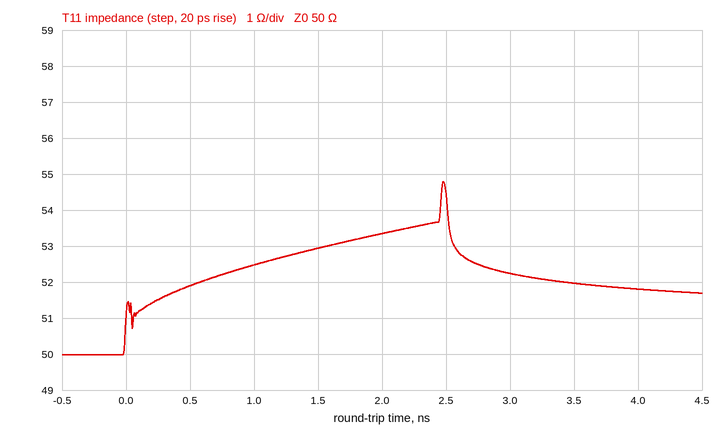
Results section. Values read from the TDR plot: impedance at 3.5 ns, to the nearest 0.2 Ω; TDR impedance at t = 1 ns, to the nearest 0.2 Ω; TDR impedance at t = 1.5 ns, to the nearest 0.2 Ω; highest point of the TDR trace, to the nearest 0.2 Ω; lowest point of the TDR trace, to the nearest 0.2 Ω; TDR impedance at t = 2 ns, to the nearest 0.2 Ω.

52.0 Ω
52.4 Ω
53.0 Ω
54.8 Ω
50.0 Ω
53.4 Ω
